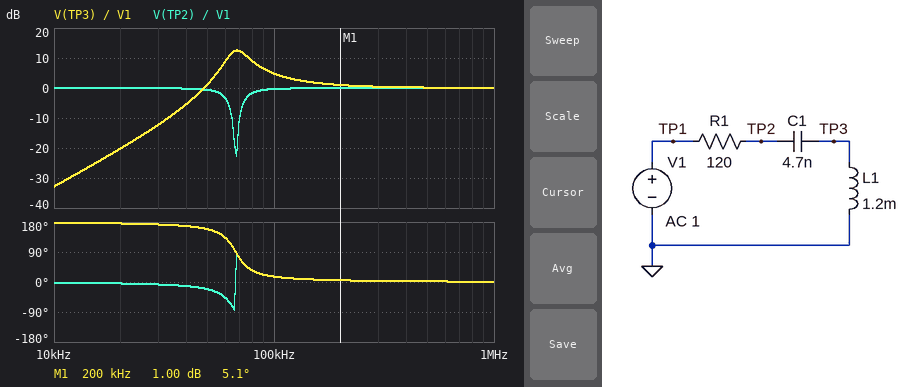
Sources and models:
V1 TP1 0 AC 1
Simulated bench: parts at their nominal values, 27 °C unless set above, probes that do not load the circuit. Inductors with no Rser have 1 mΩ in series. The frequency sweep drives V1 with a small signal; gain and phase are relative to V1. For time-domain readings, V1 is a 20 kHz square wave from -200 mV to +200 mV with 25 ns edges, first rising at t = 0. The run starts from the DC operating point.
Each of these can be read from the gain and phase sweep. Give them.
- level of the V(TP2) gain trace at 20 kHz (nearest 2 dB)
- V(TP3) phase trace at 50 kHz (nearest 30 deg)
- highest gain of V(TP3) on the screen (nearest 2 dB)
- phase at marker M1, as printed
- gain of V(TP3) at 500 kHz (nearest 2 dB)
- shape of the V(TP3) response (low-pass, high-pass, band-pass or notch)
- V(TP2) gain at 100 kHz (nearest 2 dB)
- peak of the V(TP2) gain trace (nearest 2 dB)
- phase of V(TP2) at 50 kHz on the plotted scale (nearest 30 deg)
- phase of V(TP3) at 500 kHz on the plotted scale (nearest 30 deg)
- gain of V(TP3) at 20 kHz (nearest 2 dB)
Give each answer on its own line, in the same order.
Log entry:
0 dB
150 deg
12 dB
5.1 deg
0 dB
high-pass
0 dB
0 dB
-30 deg
0 deg
-20 dB
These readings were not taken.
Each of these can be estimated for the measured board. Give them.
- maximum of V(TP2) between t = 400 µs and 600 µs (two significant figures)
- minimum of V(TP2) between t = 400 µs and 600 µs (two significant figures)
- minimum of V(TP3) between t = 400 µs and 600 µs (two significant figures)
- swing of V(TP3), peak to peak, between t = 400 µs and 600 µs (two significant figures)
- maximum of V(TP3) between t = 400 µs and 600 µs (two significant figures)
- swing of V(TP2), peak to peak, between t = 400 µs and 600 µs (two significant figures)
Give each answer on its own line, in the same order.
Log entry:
260 mV
-260 mV
-420 mV
840 mV
420 mV
530 mV
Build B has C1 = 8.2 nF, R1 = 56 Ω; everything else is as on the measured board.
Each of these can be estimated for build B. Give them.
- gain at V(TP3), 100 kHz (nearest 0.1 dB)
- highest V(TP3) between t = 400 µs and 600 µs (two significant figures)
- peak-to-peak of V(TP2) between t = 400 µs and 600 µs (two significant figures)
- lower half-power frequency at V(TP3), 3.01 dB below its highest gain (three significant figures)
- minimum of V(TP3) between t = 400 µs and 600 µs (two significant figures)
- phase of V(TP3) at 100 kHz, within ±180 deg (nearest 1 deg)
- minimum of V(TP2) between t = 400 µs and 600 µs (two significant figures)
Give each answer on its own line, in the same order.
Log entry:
2.5 dB
350 mV
470 mV
47.6 kHz
-350 mV
6 deg
-240 mV
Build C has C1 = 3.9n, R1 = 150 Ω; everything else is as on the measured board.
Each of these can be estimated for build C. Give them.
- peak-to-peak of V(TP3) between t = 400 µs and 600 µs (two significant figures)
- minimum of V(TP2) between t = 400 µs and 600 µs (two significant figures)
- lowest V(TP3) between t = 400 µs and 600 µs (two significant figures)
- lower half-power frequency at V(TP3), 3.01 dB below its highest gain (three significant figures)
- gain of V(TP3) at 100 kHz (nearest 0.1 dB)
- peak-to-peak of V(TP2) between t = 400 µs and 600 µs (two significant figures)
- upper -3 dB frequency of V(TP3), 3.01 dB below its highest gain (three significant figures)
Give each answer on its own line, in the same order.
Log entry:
690 mV
-250 mV
-350 mV
66.3 kHz
6.0 dB
510 mV
88.2 kHz
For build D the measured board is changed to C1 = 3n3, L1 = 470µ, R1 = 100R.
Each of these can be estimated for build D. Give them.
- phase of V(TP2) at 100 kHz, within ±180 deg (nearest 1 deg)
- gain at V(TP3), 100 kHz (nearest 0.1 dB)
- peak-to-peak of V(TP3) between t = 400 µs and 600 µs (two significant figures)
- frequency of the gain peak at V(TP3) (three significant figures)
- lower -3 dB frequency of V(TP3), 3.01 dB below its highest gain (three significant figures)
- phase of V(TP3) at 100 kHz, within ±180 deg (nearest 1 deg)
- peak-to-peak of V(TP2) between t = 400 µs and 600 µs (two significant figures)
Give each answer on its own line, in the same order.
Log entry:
-28 deg
2.9 dB
770 mV
130 kHz
115 kHz
152 deg
510 mV
